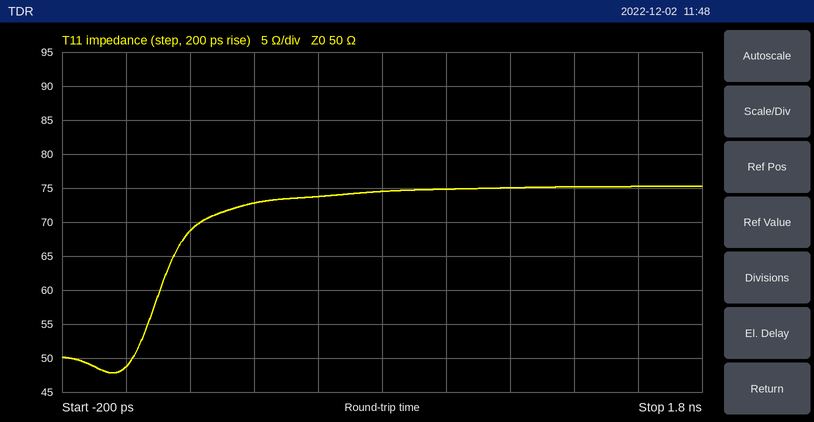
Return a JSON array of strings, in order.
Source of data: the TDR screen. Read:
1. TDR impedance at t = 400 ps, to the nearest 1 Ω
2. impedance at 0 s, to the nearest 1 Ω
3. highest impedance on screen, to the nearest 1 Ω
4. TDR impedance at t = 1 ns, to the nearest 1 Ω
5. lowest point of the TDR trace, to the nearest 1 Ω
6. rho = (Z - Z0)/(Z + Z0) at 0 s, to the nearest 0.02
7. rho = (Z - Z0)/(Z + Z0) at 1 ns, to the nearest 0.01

["73 Ω", "49 Ω", "75 Ω", "75 Ω", "48 Ω", "-0.02", "+0.20"]
